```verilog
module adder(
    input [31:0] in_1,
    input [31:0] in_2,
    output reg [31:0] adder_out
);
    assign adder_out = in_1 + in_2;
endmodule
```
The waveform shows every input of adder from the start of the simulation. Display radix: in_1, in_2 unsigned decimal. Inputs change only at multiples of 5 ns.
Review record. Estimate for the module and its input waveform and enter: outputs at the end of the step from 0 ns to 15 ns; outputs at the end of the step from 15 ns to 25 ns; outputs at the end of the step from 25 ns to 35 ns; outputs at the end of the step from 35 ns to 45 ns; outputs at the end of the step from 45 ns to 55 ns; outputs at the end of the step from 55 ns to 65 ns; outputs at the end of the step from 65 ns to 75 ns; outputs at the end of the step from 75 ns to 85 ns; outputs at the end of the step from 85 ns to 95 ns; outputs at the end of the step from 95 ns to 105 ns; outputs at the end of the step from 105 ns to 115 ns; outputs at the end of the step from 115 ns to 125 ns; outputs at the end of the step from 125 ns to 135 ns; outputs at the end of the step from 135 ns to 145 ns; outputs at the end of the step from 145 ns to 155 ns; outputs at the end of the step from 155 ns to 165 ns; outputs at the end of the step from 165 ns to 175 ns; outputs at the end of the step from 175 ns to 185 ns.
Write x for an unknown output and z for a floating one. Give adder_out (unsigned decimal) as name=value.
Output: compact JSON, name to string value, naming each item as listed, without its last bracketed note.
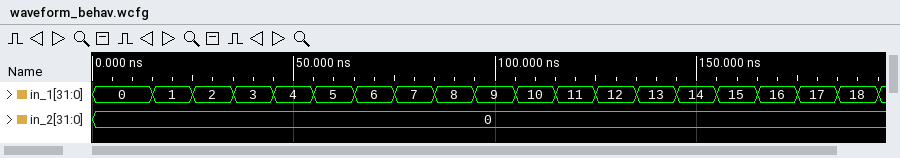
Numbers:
{"outputs at the end of the step from 0 ns to 15 ns": "adder_out=0", "outputs at the end of the step from 15 ns to 25 ns": "adder_out=1", "outputs at the end of the step from 25 ns to 35 ns": "adder_out=2", "outputs at the end of the step from 35 ns to 45 ns": "adder_out=3", "outputs at the end of the step from 45 ns to 55 ns": "adder_out=4", "outputs at the end of the step from 55 ns to 65 ns": "adder_out=5", "outputs at the end of the step from 65 ns to 75 ns": "adder_out=6", "outputs at the end of the step from 75 ns to 85 ns": "adder_out=7", "outputs at the end of the step from 85 ns to 95 ns": "adder_out=8", "outputs at the end of the step from 95 ns to 105 ns": "adder_out=9", "outputs at the end of the step from 105 ns to 115 ns": "adder_out=10", "outputs at the end of the step from 115 ns to 125 ns": "adder_out=11", "outputs at the end of the step from 125 ns to 135 ns": "adder_out=12", "outputs at the end of the step from 135 ns to 145 ns": "adder_out=13", "outputs at the end of the step from 145 ns to 155 ns": "adder_out=14", "outputs at the end of the step from 155 ns to 165 ns": "adder_out=15", "outputs at the end of the step from 165 ns to 175 ns": "adder_out=16", "outputs at the end of the step from 175 ns to 185 ns": "adder_out=17"}
